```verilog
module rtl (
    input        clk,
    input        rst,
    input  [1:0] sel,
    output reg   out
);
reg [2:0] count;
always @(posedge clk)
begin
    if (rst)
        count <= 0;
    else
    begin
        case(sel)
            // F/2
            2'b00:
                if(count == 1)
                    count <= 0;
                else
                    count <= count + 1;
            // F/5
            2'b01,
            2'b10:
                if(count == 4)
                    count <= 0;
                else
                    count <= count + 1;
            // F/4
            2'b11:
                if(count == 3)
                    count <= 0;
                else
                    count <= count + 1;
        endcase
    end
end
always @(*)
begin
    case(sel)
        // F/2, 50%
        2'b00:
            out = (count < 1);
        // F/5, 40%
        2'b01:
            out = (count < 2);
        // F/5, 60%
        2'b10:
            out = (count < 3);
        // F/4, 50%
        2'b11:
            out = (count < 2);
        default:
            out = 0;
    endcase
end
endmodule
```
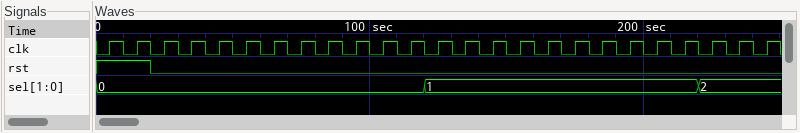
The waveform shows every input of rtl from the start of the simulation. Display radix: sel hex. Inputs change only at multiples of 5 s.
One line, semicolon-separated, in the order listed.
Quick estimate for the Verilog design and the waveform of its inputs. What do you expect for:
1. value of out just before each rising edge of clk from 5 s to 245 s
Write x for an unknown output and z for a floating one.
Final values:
x 1 1 0 1 0 1 0 1 0 1 0 1 1 0 0 0 1 1 0 0 0 1 1 1
